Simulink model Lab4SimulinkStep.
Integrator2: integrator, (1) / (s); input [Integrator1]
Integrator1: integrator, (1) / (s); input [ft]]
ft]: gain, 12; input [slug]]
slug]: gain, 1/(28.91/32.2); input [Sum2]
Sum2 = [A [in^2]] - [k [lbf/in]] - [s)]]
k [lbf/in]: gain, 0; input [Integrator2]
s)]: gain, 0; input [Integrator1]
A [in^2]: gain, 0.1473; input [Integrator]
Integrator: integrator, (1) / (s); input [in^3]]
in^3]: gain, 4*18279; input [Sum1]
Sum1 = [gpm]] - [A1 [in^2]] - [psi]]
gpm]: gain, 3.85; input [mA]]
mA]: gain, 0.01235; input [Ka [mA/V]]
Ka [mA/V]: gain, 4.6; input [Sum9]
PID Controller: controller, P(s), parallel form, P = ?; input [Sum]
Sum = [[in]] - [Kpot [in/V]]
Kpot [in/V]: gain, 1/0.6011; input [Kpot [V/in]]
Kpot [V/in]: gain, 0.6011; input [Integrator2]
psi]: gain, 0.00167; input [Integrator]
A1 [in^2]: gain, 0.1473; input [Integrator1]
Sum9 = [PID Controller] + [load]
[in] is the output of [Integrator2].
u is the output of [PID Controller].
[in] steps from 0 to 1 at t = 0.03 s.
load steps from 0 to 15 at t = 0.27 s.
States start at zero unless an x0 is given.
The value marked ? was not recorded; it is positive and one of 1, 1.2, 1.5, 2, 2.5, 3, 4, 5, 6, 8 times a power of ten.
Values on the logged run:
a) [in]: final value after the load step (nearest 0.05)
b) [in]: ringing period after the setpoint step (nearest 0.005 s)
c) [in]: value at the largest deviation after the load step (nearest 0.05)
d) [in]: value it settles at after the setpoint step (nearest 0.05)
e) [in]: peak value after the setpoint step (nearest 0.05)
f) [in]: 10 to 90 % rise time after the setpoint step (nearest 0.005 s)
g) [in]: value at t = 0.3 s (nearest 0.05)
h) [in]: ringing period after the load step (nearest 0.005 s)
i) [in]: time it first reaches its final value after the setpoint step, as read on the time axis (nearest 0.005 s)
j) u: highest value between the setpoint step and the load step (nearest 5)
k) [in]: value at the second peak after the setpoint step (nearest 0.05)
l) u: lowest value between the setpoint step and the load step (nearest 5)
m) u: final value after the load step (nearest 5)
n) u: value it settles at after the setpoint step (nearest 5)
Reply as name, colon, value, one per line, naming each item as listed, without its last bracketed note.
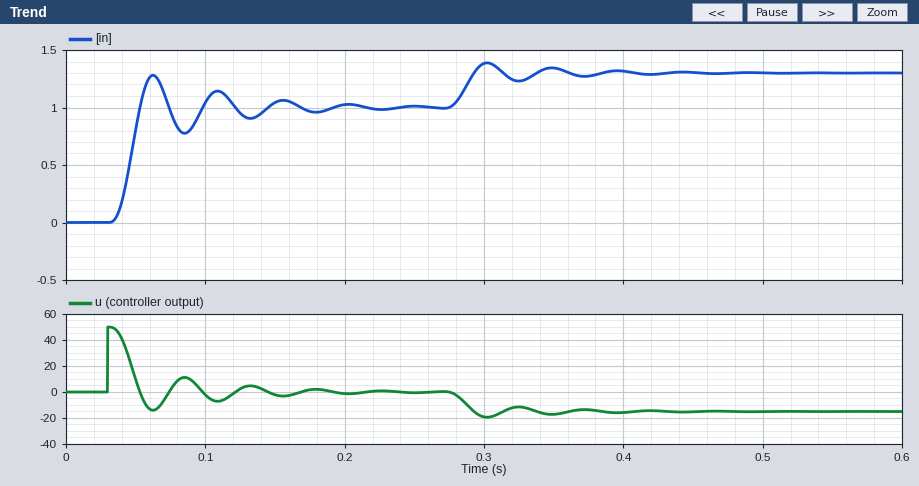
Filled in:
[in]: final value after the load step: 1.30
[in]: ringing period after the setpoint step: 0.045 s
[in]: value at the largest deviation after the load step: 1.40
[in]: value it settles at after the setpoint step: 1.00
[in]: peak value after the setpoint step: 1.30
[in]: 10 to 90 % rise time after the setpoint step: 0.015 s
[in]: value at t = 0.3 s: 1.40
[in]: ringing period after the load step: 0.045 s
[in]: time it first reaches its final value after the setpoint step, as read on the time axis: 0.055 s
u: highest value between the setpoint step and the load step: 50
[in]: value at the second peak after the setpoint step: 1.15
u: lowest value between the setpoint step and the load step: -15
u: final value after the load step: -15
u: value it settles at after the setpoint step: 0
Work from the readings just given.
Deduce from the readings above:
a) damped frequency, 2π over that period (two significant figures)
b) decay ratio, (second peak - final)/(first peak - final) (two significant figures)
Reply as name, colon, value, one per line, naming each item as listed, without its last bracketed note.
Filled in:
damped frequency, 2π over that period: 140 rad/s
decay ratio, (second peak - final)/(first peak - final): 0.50
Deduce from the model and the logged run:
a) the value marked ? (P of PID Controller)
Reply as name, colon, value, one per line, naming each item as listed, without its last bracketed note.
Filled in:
the value marked ?: 50
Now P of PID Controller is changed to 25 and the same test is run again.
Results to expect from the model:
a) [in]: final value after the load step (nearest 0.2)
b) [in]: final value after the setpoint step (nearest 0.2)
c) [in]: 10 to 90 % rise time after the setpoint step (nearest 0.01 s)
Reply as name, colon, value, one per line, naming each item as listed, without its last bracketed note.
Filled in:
[in]: final value after the load step: 1.6
[in]: final value after the setpoint step: 1.0
[in]: 10 to 90 % rise time after the setpoint step: 0.05 s
